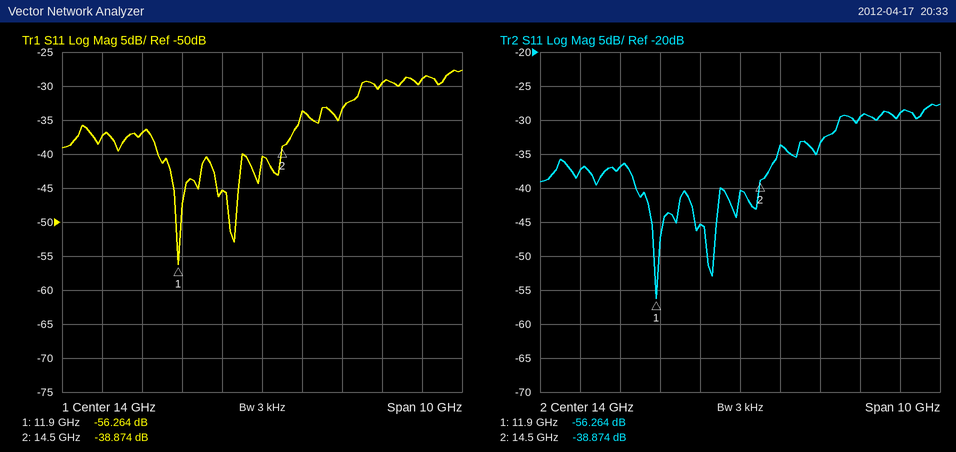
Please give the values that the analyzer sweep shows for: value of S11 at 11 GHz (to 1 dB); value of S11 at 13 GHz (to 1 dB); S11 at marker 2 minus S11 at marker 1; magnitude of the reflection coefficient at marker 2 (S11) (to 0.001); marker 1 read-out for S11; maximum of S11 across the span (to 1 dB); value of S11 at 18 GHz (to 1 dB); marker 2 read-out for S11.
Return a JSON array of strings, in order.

["-37 dB", "-45 dB", "17.390 dB", "0.011", "-56.264 dB", "-28 dB", "-29 dB", "-38.874 dB"]
